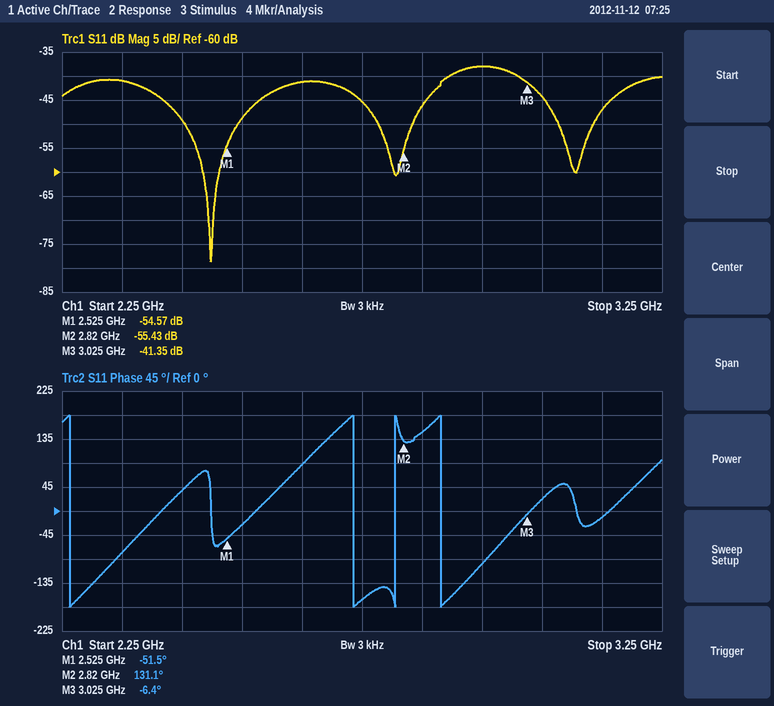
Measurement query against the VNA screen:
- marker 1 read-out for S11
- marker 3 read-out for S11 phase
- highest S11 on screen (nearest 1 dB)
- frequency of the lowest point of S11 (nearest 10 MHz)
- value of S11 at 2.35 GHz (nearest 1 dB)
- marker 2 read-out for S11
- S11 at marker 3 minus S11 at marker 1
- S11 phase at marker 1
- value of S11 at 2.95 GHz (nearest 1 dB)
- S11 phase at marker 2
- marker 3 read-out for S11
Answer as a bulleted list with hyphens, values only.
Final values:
- -54.57 dB
- -6.4°
- -38 dB
- 2.50 GHz
- -41 dB
- -55.43 dB
- 13.22 dB
- -51.5°
- -38 dB
- 131.1°
- -41.35 dB
